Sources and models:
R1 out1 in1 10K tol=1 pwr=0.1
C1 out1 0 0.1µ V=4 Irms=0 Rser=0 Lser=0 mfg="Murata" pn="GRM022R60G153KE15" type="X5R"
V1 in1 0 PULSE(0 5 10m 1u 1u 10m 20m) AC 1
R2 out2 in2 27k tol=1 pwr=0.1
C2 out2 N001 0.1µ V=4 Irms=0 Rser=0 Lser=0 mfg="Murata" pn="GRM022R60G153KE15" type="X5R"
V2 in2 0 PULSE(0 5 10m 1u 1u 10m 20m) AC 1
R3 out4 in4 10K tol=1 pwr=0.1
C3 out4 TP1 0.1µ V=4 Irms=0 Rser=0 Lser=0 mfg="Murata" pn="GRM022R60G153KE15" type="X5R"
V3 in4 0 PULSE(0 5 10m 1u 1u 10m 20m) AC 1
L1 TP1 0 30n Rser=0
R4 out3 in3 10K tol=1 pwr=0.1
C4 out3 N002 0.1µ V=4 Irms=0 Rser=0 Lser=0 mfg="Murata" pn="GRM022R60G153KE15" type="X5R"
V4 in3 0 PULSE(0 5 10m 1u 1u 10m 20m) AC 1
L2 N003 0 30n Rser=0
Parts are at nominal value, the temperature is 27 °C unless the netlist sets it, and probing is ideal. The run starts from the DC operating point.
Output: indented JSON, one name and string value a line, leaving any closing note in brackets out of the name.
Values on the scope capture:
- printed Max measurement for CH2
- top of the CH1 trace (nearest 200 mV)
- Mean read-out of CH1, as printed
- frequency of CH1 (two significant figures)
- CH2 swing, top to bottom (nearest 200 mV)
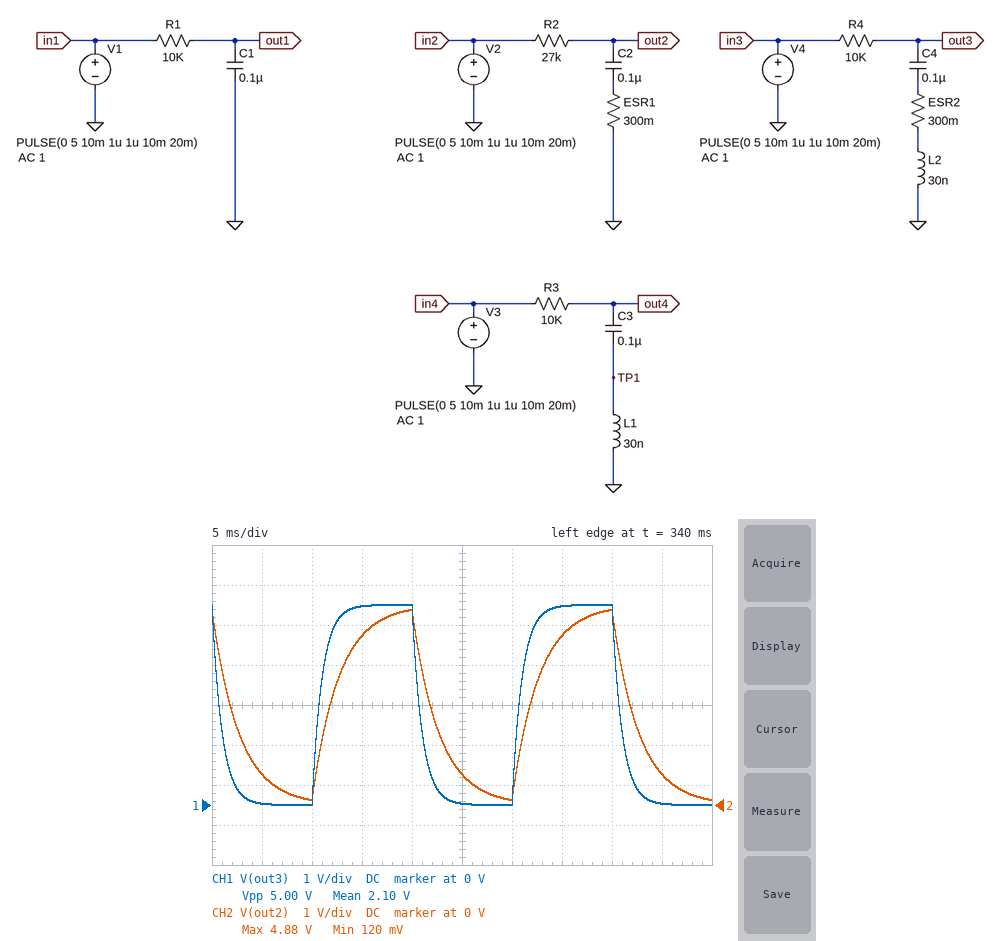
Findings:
{
  "printed Max measurement for CH2": "4.88 V",
  "top of the CH1 trace": "5.0 V",
  "Mean read-out of CH1, as printed": "2.10 V",
  "frequency of CH1": "50 Hz",
  "CH2 swing, top to bottom": "4.8 V"
}
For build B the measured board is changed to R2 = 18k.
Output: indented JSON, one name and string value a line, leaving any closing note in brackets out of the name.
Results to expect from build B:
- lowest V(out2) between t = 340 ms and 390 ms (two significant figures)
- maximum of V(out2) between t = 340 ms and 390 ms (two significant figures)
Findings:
{
  "lowest V(out2) between t = 340 ms and 390 ms": "19 mV",
  "maximum of V(out2) between t = 340 ms and 390 ms": "5.0 V"
}
